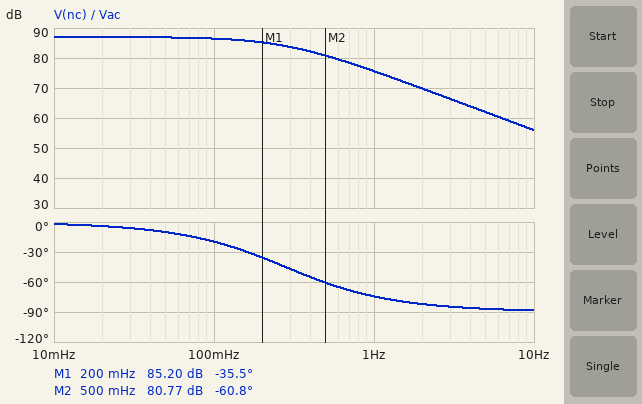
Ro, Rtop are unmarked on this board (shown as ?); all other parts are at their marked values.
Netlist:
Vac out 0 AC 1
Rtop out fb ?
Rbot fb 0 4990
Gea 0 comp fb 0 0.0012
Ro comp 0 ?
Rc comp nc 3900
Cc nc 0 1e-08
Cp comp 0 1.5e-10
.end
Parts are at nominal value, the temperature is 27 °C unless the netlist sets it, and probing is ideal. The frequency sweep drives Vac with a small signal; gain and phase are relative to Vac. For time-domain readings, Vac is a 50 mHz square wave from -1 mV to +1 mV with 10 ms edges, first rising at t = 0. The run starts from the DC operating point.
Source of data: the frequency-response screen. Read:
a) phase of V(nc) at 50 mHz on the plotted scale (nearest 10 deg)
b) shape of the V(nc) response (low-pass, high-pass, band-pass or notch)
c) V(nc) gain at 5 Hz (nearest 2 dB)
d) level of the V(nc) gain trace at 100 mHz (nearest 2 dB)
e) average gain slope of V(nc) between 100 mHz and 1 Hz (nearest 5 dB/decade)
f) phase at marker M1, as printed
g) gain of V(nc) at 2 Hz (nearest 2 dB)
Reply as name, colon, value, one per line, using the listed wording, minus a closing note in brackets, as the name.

phase of V(nc) at 50 mHz on the plotted scale: -10 deg
shape of the V(nc) response: low-pass
V(nc) gain at 5 Hz: 62 dB
level of the V(nc) gain trace at 100 mHz: 86 dB
average gain slope of V(nc) between 100 mHz and 1 Hz: -10 dB/decade
phase at marker M1, as printed: -35.5 deg
gain of V(nc) at 2 Hz: 70 dB
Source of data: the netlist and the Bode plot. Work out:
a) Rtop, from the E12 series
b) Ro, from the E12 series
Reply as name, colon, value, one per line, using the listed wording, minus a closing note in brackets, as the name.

Rtop, from the E12 series: 10 kΩ
Ro, from the E12 series: 56 MΩ
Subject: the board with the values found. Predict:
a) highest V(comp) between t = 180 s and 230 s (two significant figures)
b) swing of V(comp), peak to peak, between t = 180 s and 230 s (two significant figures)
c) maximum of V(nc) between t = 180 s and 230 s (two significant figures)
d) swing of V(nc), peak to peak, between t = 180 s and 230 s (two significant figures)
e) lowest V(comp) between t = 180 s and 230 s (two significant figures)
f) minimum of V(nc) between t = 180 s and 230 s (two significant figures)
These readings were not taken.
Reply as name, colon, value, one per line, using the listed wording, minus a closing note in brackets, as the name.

highest V(comp) between t = 180 s and 230 s: 22 V
swing of V(comp), peak to peak, between t = 180 s and 230 s: 45 V
maximum of V(nc) between t = 180 s and 230 s: 22 V
swing of V(nc), peak to peak, between t = 180 s and 230 s: 45 V
lowest V(comp) between t = 180 s and 230 s: -22 V
minimum of V(nc) between t = 180 s and 230 s: -22 V
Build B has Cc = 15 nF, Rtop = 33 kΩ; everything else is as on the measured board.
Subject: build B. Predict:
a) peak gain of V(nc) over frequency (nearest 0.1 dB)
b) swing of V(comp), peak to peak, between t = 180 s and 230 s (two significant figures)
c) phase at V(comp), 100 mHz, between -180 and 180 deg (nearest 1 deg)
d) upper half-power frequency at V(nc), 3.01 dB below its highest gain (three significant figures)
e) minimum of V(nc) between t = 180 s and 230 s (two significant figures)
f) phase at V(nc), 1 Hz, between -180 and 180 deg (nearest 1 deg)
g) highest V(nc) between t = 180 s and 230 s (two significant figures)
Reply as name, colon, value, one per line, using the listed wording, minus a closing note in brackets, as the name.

peak gain of V(nc) over frequency: 78.9 dB
swing of V(comp), peak to peak, between t = 180 s and 230 s: 18 V
phase at V(comp), 100 mHz, between -180 and 180 deg: -28 deg
upper half-power frequency at V(nc), 3.01 dB below its highest gain: 188 mHz
minimum of V(nc) between t = 180 s and 230 s: -8.8 V
phase at V(nc), 1 Hz, between -180 and 180 deg: -79 deg
highest V(nc) between t = 180 s and 230 s: 8.8 V
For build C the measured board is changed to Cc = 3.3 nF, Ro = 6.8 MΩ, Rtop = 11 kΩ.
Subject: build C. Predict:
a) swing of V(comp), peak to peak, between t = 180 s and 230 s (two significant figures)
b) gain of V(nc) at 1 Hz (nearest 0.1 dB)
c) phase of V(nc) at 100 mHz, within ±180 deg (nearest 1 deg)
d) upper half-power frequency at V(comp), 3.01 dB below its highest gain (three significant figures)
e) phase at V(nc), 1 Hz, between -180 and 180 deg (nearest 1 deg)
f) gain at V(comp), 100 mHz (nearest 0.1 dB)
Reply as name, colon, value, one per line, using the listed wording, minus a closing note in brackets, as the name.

swing of V(comp), peak to peak, between t = 180 s and 230 s: 5.1 V
gain of V(nc) at 1 Hz: 68.0 dB
phase of V(nc) at 100 mHz, within ±180 deg: -1 deg
upper half-power frequency at V(comp), 3.01 dB below its highest gain: 6.78 Hz
phase at V(nc), 1 Hz, between -180 and 180 deg: -8 deg
gain at V(comp), 100 mHz: 68.1 dB
